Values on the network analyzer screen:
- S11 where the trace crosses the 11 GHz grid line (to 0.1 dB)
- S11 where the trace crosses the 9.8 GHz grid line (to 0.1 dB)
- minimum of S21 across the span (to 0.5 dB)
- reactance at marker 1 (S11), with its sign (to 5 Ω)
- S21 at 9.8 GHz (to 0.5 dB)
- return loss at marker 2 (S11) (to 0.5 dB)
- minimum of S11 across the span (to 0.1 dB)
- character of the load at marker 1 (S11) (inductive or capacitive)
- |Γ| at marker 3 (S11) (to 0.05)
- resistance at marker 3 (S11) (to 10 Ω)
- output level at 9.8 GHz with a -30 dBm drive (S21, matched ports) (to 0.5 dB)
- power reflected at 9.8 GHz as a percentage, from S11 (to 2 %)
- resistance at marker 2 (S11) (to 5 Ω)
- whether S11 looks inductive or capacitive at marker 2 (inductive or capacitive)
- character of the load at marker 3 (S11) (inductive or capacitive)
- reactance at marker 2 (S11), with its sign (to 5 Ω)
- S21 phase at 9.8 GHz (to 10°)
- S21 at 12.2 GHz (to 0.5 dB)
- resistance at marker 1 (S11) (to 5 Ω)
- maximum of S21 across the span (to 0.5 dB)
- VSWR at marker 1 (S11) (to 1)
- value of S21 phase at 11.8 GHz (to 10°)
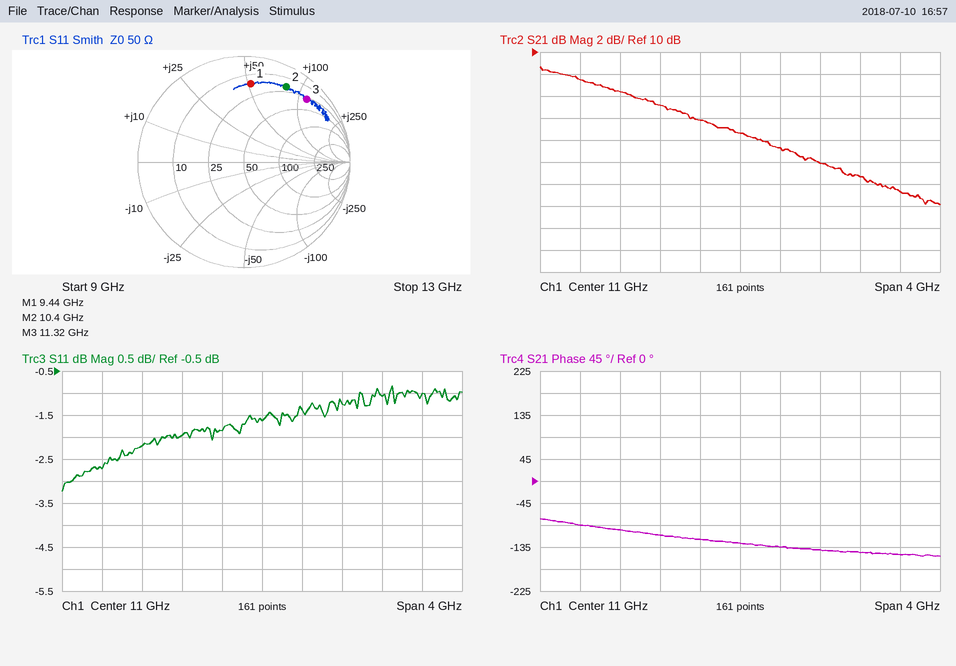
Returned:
-1.6 dB
-2.2 dB
-4.0 dB
+50 Ω
6.5 dB
2.0 dB
-3.2 dB
inductive
0.85
30 Ω
-23.5 dBm
60 %
20 Ω
inductive
inductive
+80 Ω
-100°
-1.5 dB
15 Ω
8.5 dB
7
-140°
